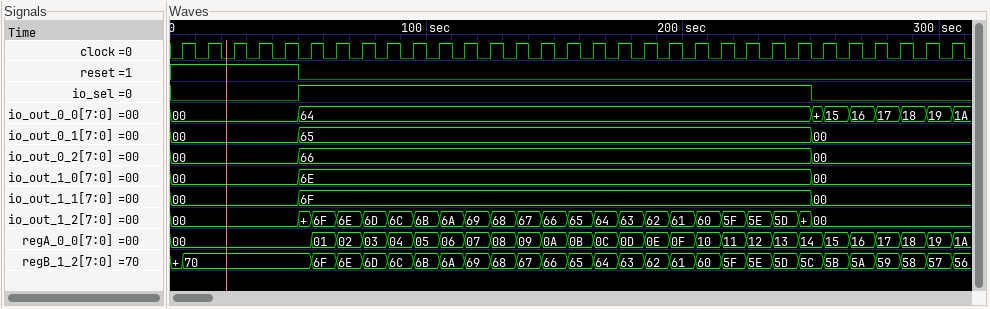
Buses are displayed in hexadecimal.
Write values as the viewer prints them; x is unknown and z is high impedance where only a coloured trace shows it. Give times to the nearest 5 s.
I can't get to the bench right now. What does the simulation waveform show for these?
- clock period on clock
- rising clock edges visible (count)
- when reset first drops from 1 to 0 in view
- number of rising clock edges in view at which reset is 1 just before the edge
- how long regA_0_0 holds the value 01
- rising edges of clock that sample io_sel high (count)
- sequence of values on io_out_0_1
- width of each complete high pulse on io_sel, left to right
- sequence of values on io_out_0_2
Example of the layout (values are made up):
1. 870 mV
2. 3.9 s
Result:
1. 10 s
2. 31
3. 50 s
4. 5
5. 10 s
6. 20
7. 00, 65, 00
8. 200 s
9. 00, 66, 00
